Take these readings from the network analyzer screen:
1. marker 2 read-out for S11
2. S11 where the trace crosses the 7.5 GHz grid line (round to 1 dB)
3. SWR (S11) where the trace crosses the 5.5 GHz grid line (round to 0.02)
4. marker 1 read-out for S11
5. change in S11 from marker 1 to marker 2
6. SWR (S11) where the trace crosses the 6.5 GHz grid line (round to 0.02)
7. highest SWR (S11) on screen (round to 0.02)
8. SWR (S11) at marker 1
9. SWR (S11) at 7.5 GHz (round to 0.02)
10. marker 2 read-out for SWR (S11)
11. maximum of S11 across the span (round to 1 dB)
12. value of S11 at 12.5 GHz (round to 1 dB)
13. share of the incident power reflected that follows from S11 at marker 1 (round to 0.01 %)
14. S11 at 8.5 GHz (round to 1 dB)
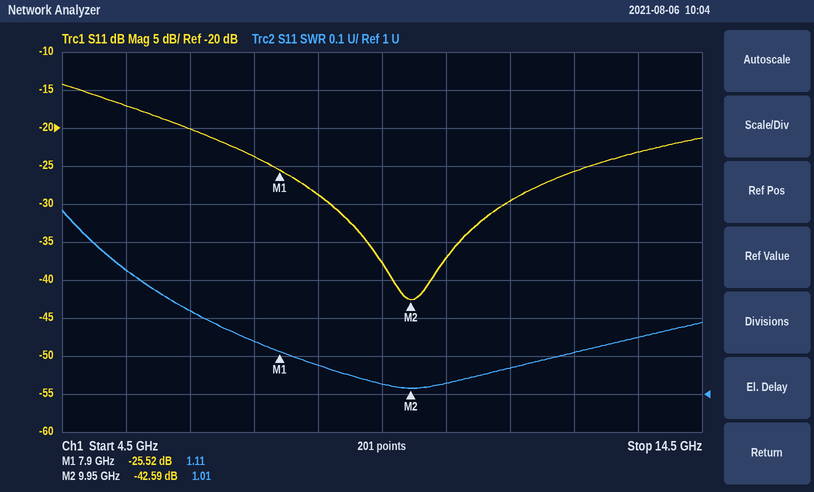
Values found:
-42.59 dB
-24 dB
1.32
-25.52 dB
-17.07 dB
1.22
1.48
1.11
1.14
1.01
-14 dB
-26 dB
0.28 %
-29 dB
